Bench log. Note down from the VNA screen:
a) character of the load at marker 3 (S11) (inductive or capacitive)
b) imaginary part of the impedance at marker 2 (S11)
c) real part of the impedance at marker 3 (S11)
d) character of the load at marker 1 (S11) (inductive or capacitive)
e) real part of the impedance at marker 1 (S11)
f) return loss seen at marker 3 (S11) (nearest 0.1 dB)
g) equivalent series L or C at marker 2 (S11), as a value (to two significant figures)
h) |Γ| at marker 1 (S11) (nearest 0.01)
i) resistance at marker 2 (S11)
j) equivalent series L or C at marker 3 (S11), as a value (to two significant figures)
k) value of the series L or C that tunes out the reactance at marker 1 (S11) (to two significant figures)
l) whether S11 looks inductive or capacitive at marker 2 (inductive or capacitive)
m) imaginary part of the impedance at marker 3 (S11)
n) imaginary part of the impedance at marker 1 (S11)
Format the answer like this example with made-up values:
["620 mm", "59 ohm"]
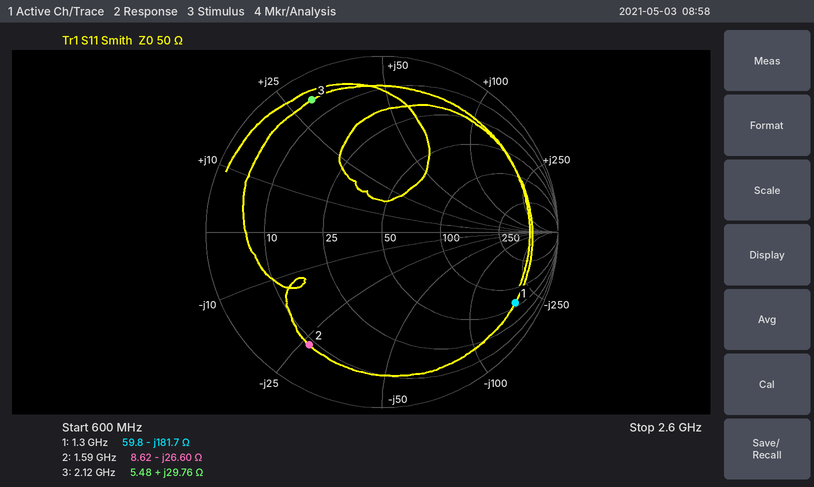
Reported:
["inductive", "-26.60 Ω", "5.48 Ω", "capacitive", "59.8 Ω", "1.4 dB", "3.8 pF", "0.86", "8.62 Ω", "2.2 nH", "22 nH", "capacitive", "+29.76 Ω", "-181.7 Ω"]
